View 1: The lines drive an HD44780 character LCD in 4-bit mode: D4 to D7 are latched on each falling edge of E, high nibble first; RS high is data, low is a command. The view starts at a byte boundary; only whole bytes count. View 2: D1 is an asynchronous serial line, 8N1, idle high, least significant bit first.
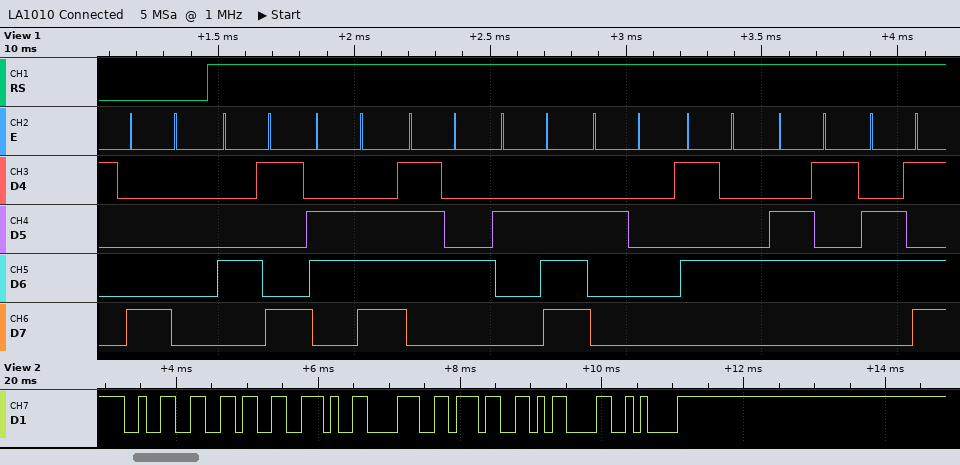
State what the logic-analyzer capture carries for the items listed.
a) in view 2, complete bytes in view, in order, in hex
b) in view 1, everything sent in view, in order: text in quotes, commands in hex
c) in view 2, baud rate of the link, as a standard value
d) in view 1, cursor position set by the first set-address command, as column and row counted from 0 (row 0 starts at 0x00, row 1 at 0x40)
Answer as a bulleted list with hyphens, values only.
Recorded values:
- 32 36 2E 38 37 0D 0A
- 0x80 "Int. Tem"
- 9600 baud
- column 0, row 0
